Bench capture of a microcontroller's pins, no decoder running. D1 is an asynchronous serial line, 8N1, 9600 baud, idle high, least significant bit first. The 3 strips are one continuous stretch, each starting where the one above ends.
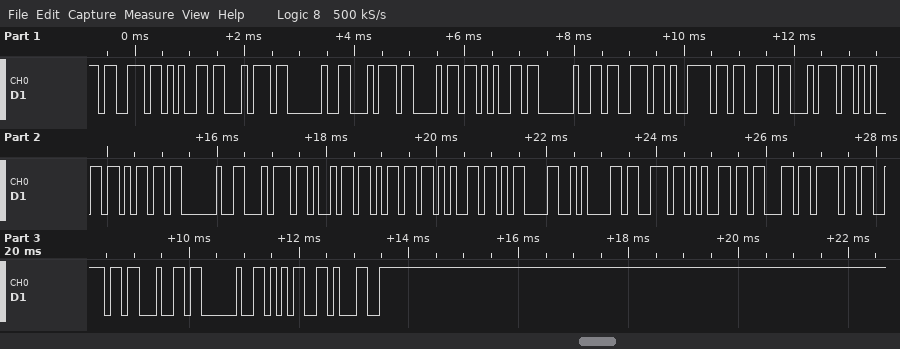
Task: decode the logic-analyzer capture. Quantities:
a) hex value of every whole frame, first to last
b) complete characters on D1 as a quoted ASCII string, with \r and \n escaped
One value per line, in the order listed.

73 65 74 20 74 68 65 20 73 79 73 74 65 6D 20 74 69 6D 65 0D 0A 73 65 63 6F 6E 64 20 35 31
"set the system time\r\nsecond 51"
